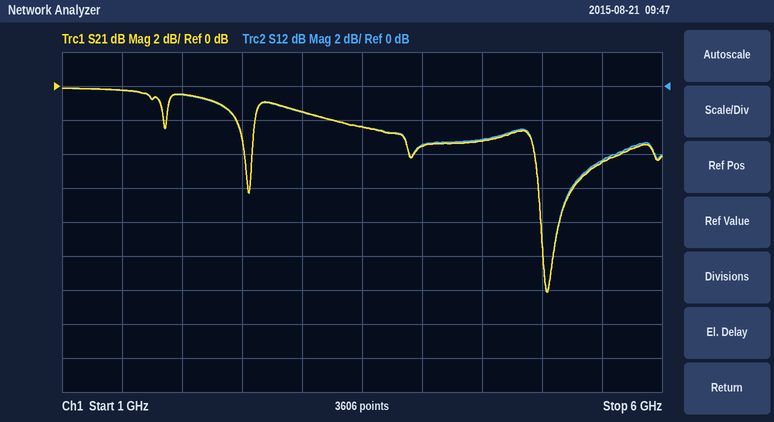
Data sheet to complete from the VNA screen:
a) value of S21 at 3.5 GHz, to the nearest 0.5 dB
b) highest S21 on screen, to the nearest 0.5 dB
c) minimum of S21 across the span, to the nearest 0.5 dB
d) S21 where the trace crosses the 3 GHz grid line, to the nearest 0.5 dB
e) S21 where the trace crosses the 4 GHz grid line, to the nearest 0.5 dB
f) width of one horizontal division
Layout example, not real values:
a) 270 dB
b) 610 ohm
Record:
a) -2.5 dB
b) 0.0 dB
c) -12.0 dB
d) -1.5 dB
e) -3.5 dB
f) 500 MHz
